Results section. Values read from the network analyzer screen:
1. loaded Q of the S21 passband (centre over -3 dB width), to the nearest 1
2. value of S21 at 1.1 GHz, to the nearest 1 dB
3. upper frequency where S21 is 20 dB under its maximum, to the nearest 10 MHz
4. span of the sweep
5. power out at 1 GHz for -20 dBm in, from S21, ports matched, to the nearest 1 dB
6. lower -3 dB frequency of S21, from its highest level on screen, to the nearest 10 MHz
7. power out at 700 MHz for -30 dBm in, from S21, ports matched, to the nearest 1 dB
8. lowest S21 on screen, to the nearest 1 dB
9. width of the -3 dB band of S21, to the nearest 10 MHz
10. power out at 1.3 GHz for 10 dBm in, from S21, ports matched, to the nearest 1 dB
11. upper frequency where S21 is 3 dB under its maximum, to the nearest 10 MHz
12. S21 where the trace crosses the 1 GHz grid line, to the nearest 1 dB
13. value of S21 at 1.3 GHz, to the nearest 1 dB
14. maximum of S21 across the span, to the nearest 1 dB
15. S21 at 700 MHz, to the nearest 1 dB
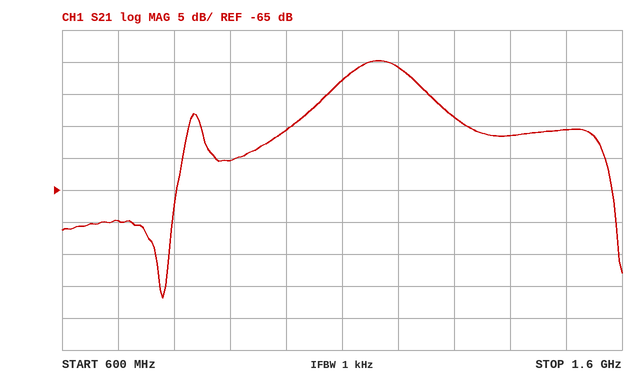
9
-48 dB
1.58 GHz
1 GHz
-76 dBm
1.10 GHz
-100 dBm
-82 dB
130 MHz
-44 dBm
1.23 GHz
-56 dB
-54 dB
-45 dB
-70 dB
